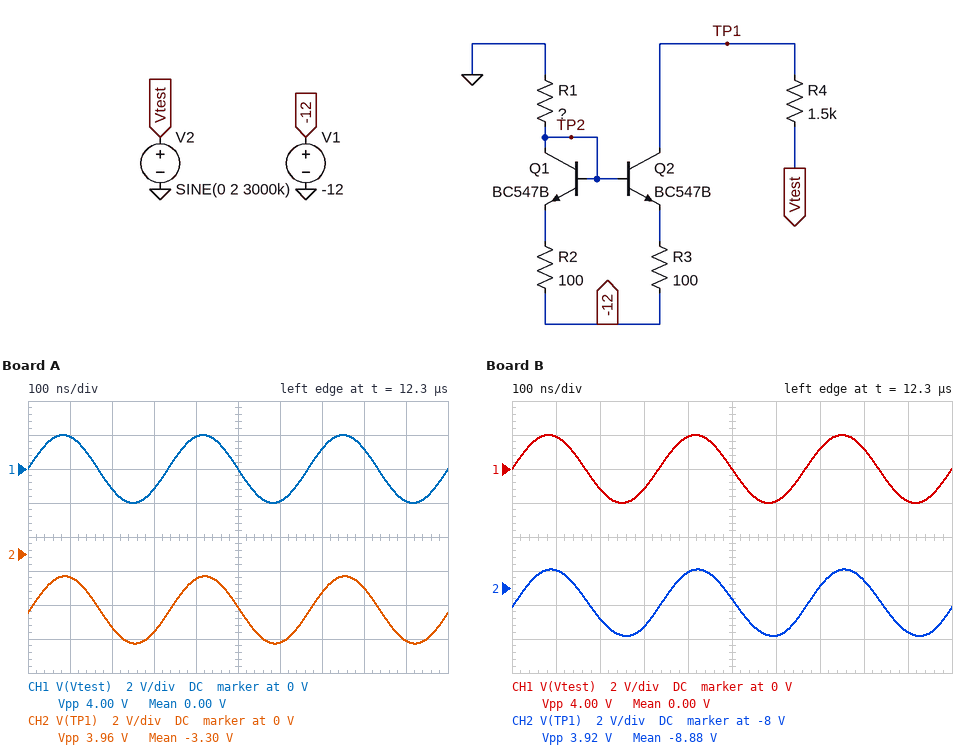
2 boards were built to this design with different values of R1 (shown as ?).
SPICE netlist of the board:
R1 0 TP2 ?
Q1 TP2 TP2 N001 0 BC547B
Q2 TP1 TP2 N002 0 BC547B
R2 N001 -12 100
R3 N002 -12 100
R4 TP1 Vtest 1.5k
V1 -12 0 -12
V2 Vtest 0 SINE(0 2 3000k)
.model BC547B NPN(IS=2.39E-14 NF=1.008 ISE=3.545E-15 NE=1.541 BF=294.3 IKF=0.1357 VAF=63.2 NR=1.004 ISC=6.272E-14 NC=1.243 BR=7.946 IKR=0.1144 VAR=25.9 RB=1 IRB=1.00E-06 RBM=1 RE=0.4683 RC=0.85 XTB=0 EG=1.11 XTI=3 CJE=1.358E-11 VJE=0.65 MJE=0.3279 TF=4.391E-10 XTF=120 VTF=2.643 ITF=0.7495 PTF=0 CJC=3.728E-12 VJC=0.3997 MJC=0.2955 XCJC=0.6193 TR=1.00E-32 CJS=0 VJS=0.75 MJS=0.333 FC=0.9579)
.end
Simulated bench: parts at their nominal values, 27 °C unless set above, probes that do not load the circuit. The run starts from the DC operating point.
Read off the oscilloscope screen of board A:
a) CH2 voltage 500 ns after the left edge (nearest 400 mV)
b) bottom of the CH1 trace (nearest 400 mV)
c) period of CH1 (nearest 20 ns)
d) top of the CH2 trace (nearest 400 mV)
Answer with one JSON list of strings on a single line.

["-3.2 V", "-2.0 V", "340 ns", "-1.2 V"]
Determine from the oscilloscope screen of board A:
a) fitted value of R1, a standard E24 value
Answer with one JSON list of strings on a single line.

["5.1 kΩ"]
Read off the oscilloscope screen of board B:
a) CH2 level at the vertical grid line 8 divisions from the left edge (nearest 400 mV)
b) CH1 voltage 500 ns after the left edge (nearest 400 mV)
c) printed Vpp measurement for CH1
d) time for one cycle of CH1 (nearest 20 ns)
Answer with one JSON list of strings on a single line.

["-7.6 V", "0 V", "4.00 V", "340 ns"]
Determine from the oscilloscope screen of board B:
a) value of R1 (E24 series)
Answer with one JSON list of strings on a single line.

["1.8 kΩ"]
